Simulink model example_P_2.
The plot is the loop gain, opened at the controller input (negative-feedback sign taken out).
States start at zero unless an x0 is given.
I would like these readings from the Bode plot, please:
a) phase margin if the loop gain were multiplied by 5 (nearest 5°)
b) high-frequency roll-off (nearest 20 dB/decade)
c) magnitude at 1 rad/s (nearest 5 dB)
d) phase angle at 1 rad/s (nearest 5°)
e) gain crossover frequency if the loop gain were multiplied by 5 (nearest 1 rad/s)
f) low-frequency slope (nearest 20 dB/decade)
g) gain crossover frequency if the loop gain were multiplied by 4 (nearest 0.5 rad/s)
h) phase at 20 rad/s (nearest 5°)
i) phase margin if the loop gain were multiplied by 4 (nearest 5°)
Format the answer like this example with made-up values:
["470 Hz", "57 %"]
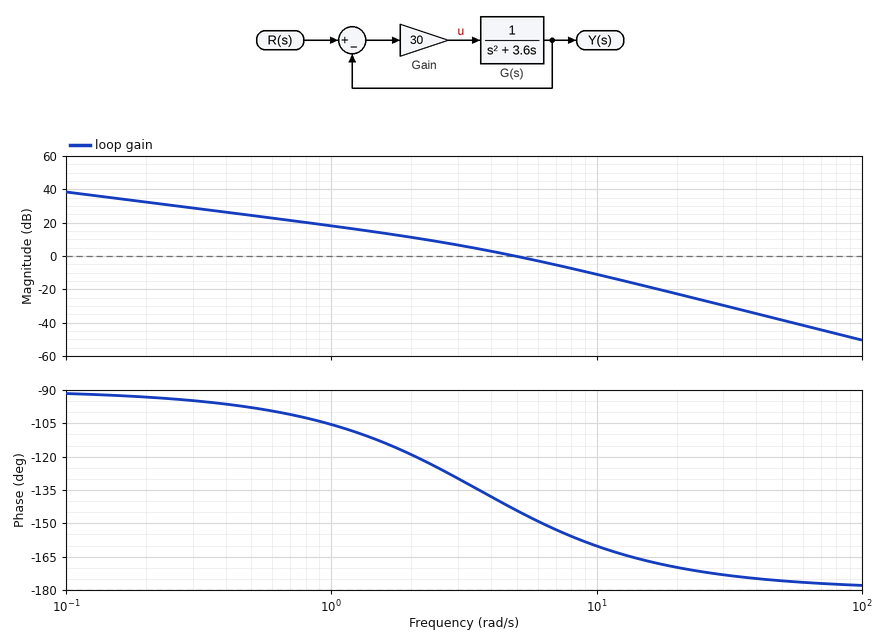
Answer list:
["15°", "-40 dB/decade", "20 dB", "-105°", "12 rad/s", "-20 dB/decade", "10.5 rad/s", "-170°", "20°"]
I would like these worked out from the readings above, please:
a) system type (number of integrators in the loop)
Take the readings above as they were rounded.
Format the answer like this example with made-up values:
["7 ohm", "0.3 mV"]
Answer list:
["1"]
